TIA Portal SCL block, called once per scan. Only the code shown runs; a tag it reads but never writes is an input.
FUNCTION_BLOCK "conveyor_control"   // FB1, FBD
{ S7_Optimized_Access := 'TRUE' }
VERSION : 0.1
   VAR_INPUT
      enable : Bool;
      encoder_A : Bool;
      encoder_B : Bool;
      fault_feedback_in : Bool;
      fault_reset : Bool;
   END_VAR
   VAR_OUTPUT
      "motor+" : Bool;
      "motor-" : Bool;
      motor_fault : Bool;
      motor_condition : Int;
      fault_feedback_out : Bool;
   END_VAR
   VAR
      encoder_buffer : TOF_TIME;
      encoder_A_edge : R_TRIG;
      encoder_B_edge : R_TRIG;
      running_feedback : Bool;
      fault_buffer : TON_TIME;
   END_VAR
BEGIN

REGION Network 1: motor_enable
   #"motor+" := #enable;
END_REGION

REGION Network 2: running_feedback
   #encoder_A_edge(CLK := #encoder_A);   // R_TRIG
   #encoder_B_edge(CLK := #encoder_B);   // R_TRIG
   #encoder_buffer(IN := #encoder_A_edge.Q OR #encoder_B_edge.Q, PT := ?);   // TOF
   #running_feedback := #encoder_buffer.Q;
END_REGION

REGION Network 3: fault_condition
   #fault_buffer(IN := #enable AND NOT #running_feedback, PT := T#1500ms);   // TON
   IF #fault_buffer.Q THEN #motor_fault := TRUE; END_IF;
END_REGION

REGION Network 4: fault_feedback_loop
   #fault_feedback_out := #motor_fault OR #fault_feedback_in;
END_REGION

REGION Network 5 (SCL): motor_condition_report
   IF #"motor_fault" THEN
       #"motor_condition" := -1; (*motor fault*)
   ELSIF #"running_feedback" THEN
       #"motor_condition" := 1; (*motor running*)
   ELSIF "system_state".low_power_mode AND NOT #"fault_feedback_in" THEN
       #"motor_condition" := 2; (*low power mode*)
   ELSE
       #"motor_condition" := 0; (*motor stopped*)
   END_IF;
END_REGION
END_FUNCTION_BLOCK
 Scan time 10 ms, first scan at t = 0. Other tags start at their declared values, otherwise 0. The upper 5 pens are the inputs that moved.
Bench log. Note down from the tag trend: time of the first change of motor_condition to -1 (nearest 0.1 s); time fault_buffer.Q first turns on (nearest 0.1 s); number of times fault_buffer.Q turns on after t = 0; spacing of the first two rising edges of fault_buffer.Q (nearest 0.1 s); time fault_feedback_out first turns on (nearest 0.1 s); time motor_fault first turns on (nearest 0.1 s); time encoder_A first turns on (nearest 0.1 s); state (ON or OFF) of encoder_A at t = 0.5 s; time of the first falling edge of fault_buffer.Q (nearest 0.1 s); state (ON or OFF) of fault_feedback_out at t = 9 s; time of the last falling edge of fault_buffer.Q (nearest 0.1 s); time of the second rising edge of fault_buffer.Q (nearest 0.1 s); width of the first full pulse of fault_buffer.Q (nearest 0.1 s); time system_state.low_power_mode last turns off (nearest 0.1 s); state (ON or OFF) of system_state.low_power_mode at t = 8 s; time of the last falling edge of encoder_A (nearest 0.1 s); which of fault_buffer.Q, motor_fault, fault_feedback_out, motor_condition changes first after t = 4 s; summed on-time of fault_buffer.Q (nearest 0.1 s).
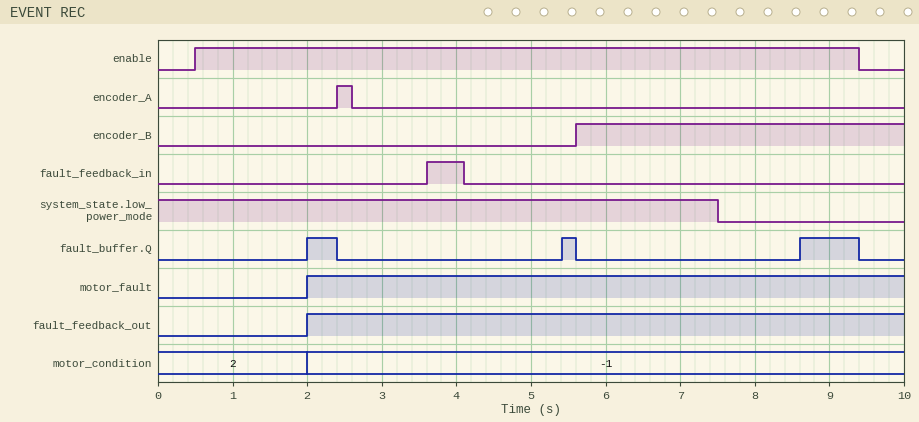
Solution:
2.0 s
2.0 s
3
3.4 s
2.0 s
2.0 s
2.4 s
OFF
2.4 s
ON
9.4 s
5.4 s
0.4 s
7.5 s
OFF
2.6 s
fault_buffer.Q
1.4 s
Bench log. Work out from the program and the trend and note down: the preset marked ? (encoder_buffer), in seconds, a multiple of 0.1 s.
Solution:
1.5 s
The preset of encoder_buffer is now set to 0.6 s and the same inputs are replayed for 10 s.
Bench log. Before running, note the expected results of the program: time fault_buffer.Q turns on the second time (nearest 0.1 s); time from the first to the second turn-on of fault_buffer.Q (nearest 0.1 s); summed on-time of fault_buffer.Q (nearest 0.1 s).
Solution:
4.5 s
2.5 s
3.2 s
